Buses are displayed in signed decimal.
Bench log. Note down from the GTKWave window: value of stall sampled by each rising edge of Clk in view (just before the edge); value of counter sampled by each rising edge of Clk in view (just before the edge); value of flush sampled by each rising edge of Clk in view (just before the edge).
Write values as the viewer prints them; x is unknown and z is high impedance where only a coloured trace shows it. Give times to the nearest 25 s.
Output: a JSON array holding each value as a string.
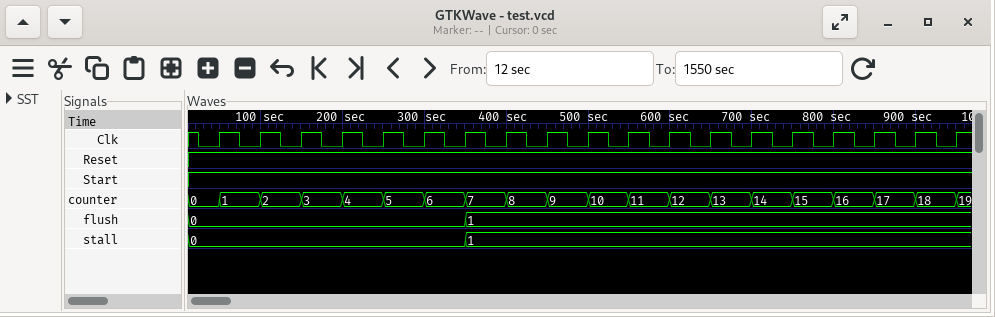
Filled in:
["0, 0, 0, 0, 0, 0, 0, 1, 1, 1, 1, 1, 1, 1, 1, 1, 1, 1, 1", "0, 1, 2, 3, 4, 5, 6, 7, 8, 9, 10, 11, 12, 13, 14, 15, 16, 17, 18", "0, 0, 0, 0, 0, 0, 0, 1, 1, 1, 1, 1, 1, 1, 1, 1, 1, 1, 1"]
